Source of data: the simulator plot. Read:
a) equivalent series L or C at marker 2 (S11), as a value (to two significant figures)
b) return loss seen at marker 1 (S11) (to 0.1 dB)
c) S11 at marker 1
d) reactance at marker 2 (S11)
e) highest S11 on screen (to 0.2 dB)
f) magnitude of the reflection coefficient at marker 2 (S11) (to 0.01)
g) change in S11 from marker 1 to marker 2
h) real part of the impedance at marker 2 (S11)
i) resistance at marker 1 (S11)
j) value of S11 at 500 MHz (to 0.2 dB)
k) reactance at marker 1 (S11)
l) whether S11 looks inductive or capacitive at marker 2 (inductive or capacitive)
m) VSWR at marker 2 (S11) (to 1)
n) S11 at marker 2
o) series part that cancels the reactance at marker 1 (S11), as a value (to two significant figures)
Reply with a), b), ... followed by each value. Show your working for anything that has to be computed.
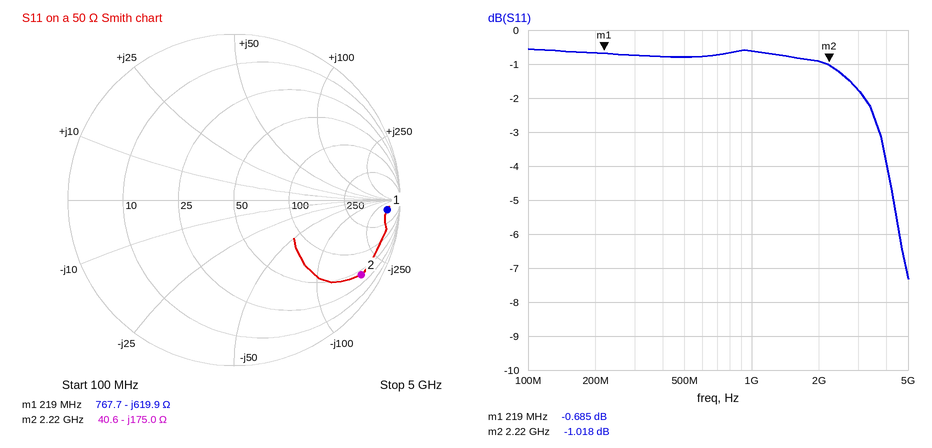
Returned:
a) C = 1/(2π × 2.22 GHz × 175 Ω) ≈ 410 fF
b) 0.7 dB
c) -0.685 dB
d) -175.0 Ω
e) -0.6 dB
f) 10^(-1.018/20) ≈ 0.89
g) -1.018 − (-0.685) = -0.333 dB
h) 40.6 Ω
i) 767.7 Ω
j) -0.8 dB
k) -619.9 Ω
l) capacitive
m) 17
n) -1.018 dB
o) L = 619.9 Ω/(2π × 219 MHz) ≈ 451 nH, so 450 nH to two significant figures
